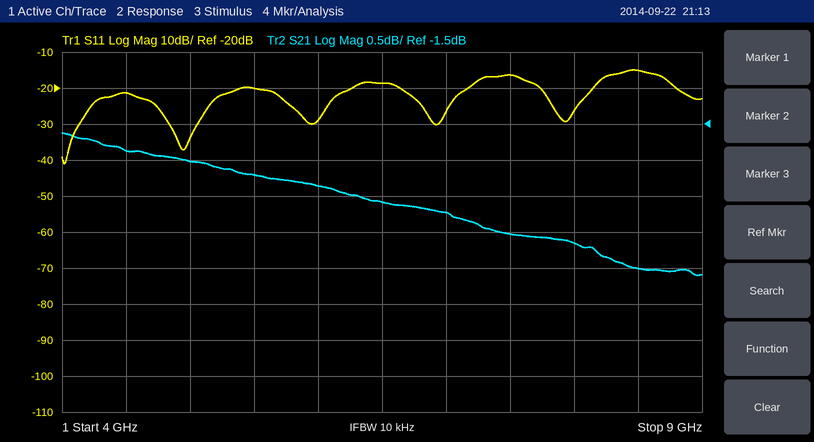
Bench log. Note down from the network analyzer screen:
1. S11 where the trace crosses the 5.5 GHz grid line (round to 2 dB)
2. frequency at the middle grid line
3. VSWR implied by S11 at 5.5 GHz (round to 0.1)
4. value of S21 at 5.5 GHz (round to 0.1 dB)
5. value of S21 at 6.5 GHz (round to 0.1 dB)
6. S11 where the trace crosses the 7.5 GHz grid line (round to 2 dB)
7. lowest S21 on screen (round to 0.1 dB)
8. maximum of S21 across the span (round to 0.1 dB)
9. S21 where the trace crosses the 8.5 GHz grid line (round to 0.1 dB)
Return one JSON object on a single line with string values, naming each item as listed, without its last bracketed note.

{"S11 where the trace crosses the 5.5 GHz grid line": "-20 dB", "frequency at the middle grid line": "6.5 GHz", "VSWR implied by S11 at 5.5 GHz": "1.2", "value of S21 at 5.5 GHz": "-2.2 dB", "value of S21 at 6.5 GHz": "-2.6 dB", "S11 where the trace crosses the 7.5 GHz grid line": "-16 dB", "lowest S21 on screen": "-3.6 dB", "maximum of S21 across the span": "-1.6 dB", "S21 where the trace crosses the 8.5 GHz grid line": "-3.5 dB"}
